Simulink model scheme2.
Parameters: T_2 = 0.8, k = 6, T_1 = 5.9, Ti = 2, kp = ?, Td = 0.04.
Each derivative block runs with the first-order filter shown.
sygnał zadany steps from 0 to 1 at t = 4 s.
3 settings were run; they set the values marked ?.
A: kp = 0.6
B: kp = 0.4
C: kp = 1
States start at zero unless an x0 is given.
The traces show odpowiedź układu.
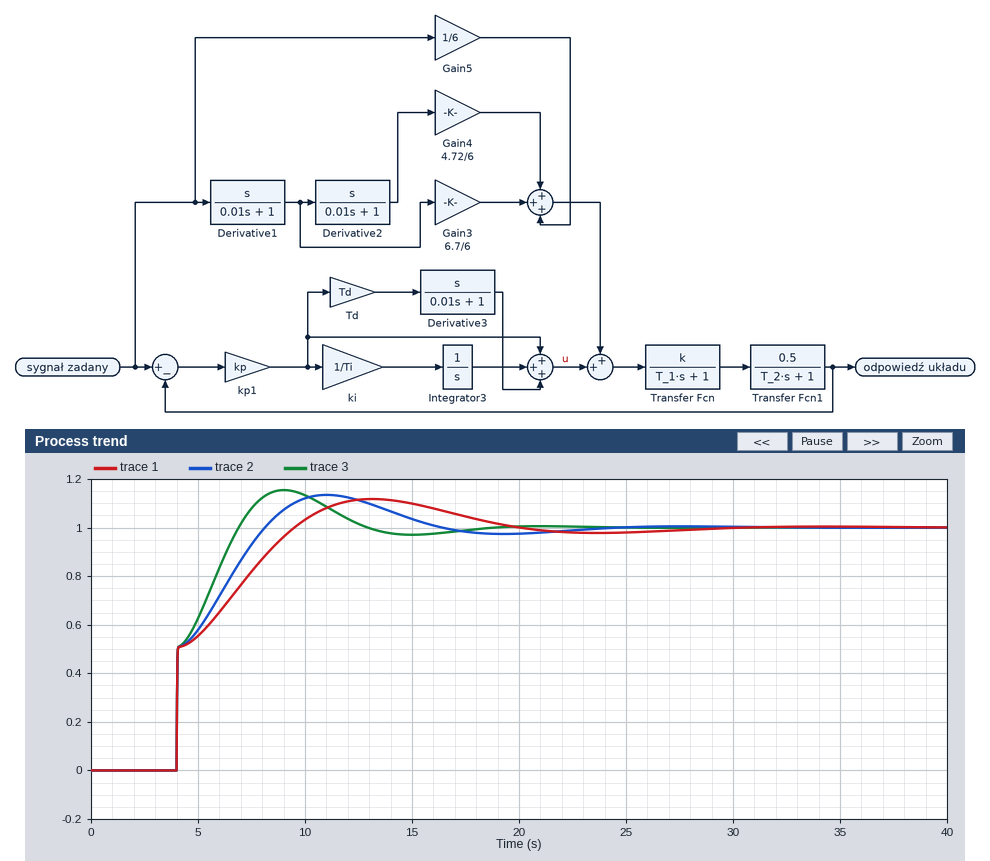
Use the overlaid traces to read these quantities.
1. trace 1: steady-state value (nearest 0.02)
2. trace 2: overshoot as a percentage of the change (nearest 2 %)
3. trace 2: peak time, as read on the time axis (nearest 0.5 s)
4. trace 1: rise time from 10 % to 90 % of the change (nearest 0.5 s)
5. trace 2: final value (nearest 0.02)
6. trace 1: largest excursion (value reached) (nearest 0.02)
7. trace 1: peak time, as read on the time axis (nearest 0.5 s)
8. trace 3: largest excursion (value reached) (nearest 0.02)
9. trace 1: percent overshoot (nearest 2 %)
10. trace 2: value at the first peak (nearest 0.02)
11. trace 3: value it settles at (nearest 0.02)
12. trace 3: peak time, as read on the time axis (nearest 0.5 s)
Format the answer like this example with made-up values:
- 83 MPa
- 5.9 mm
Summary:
- 1.00
- 14 %
- 11.0 s
- 4.5 s
- 1.00
- 1.12
- 13.0 s
- 1.16
- 12 %
- 1.14
- 1.00
- 9.0 s
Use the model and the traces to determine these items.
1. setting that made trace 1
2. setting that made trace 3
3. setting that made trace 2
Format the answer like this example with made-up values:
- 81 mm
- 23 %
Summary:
- B
- C
- A
